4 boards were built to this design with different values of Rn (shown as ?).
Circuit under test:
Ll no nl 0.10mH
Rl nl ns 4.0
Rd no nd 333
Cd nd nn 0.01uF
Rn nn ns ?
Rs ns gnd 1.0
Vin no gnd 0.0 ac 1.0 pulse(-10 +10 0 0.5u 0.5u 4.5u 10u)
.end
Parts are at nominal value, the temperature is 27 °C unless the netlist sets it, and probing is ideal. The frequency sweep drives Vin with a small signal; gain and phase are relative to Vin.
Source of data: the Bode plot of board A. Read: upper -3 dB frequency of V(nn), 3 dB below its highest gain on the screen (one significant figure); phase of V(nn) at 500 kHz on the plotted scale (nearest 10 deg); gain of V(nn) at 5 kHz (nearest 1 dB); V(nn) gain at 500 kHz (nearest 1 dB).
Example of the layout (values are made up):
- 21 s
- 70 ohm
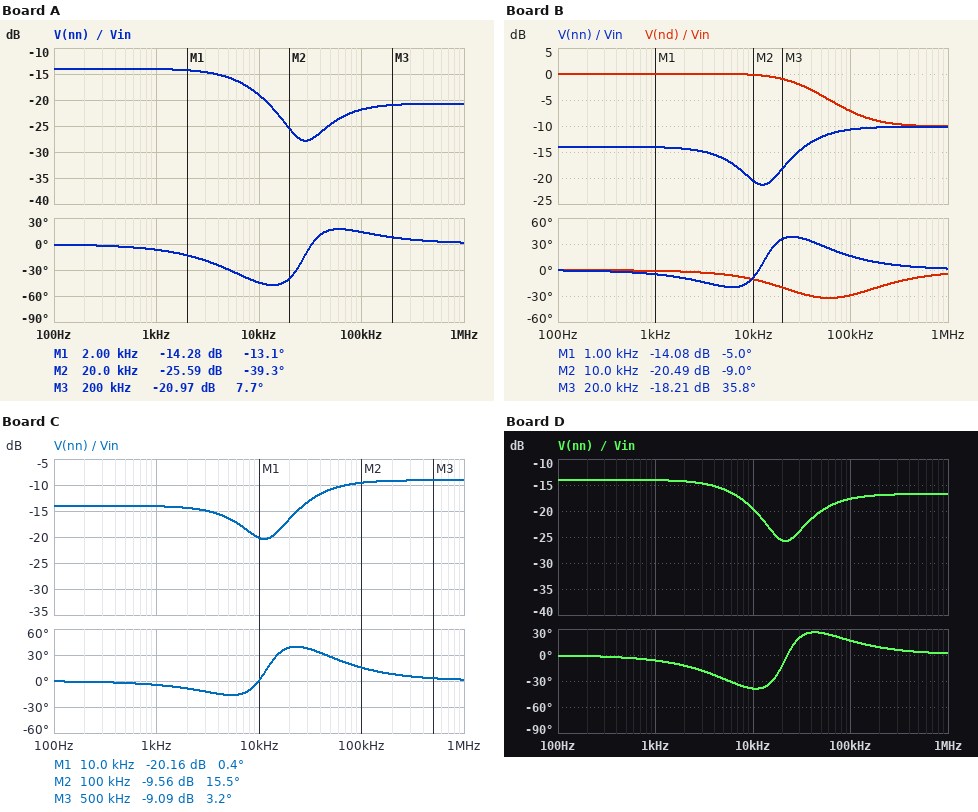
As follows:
- 7 kHz
- 0 deg
- -16 dB
- -21 dB
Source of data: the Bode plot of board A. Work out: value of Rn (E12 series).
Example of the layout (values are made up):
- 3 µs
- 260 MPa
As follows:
- 33 Ω
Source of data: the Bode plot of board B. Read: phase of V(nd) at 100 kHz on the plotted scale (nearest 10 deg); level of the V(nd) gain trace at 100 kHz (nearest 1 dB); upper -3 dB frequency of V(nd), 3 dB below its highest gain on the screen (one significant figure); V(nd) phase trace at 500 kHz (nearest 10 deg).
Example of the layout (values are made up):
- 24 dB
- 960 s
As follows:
- -30 deg
- -7 dB
- 40 kHz
- -10 deg
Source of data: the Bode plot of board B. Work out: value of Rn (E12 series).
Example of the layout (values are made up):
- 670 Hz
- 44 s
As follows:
- 150 Ω
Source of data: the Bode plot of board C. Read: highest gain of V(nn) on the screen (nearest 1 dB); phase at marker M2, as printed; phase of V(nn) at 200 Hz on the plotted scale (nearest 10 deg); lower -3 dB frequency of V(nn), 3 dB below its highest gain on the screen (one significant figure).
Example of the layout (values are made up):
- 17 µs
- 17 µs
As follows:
- -9 dB
- 15.5 deg
- 0 deg
- 40 kHz
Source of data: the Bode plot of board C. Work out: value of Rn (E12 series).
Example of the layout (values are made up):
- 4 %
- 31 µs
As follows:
- 180 Ω
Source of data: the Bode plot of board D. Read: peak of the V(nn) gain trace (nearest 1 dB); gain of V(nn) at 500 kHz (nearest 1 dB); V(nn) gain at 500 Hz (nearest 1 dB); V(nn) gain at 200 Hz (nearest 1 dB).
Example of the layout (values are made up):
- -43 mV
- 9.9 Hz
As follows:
- -14 dB
- -17 dB
- -14 dB
- -14 dB
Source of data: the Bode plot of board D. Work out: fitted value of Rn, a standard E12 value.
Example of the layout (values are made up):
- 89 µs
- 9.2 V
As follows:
- 56 Ω
